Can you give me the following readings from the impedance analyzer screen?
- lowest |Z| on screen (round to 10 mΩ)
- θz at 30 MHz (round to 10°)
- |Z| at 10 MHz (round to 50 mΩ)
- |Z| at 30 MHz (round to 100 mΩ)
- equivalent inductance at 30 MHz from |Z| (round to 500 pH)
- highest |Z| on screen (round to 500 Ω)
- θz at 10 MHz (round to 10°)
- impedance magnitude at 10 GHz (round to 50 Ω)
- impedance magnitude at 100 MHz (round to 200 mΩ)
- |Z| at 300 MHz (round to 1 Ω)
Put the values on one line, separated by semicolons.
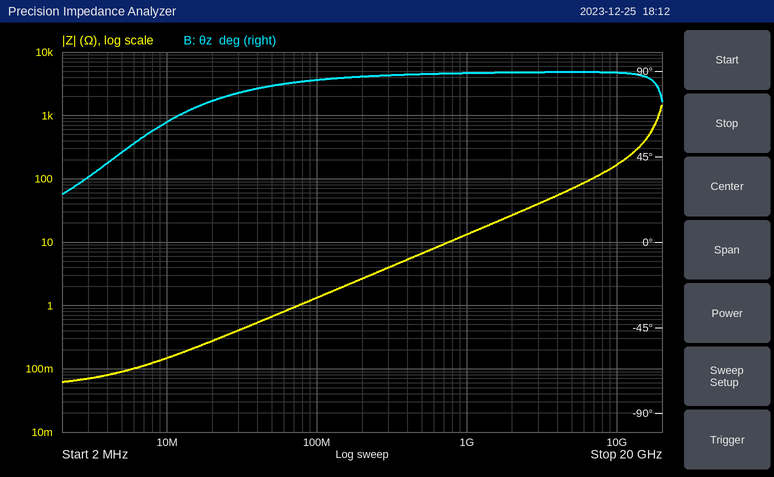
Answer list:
60 mΩ; 80°; 150 mΩ; 400 mΩ; 2.0 nH; 1.5 kΩ; 60°; 150 Ω; 1.4 Ω; 4 Ω
